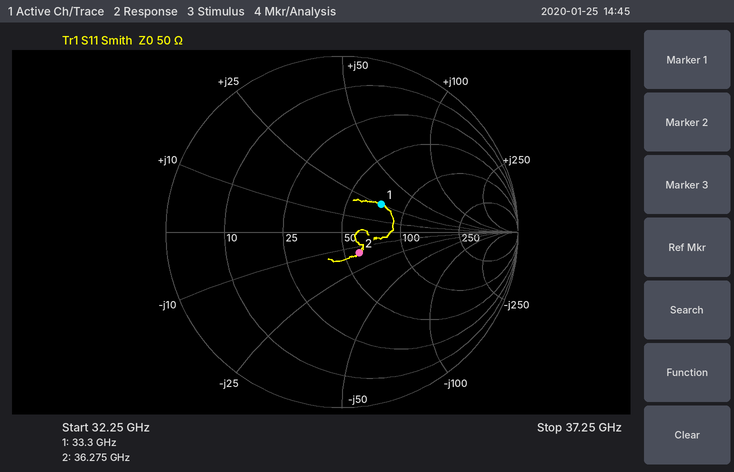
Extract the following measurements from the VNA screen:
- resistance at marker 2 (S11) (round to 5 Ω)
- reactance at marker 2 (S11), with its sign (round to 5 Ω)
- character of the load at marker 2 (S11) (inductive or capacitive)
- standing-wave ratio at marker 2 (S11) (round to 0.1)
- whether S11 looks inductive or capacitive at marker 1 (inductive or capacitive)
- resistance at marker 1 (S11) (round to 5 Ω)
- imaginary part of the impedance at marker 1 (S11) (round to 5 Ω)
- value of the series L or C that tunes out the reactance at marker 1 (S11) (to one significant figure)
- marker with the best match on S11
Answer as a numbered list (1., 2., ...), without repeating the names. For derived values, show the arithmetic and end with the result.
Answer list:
1. 60 Ω
2. -15 Ω
3. capacitive
4. 1.4
5. inductive
6. 75 Ω
7. +25 Ω
8. C = 1/(2π × 33.3 GHz × 25 Ω) ≈ 191 fF, so 200 fF to one significant figure
9. marker 2
